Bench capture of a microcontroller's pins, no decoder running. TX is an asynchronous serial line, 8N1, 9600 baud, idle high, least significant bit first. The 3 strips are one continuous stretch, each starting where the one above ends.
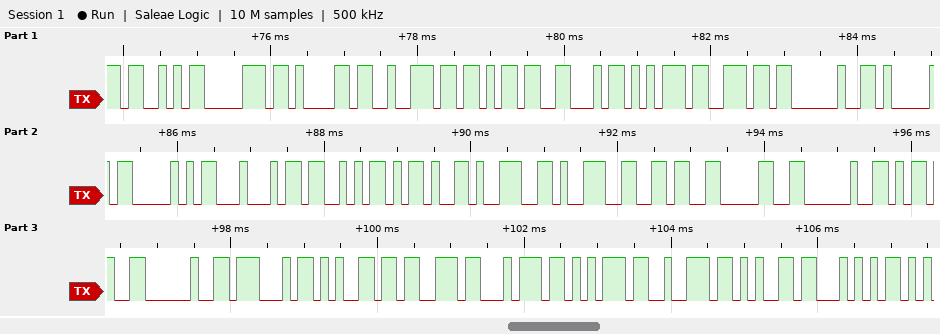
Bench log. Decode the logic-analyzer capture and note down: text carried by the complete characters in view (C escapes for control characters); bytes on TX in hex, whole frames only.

"SparkFun APDS-9960 - GestureT"
0x53 0x70 0x61 0x72 0x6B 0x46 0x75 0x6E 0x20 0x41 0x50 0x44 0x53 0x2D 0x39 0x39 0x36 0x30 0x20 0x2D 0x20 0x47 0x65 0x73 0x74 0x75 0x72 0x65 0x54
